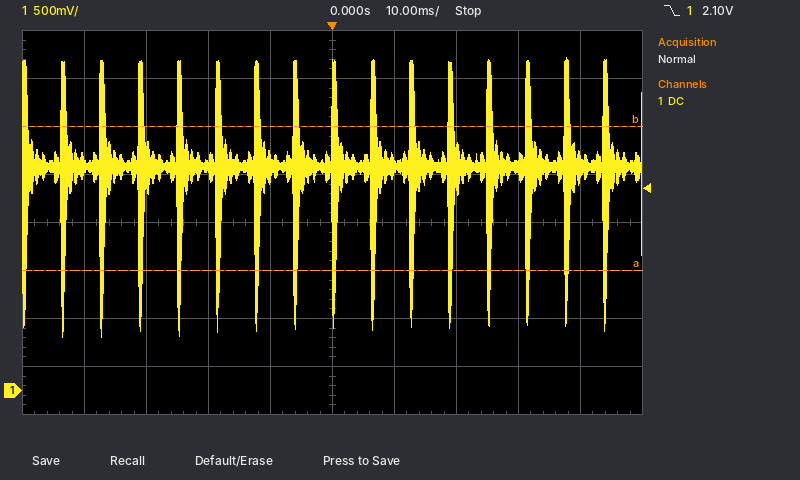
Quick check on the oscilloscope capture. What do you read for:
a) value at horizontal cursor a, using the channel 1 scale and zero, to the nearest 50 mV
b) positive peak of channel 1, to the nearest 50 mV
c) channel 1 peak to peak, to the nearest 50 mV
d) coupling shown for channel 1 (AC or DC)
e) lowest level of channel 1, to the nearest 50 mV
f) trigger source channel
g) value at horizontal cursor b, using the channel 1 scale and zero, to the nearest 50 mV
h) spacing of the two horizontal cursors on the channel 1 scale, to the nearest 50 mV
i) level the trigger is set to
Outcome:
1.25 V
3.45 V
2.90 V
DC
550 mV
channel 1
2.75 V
1.50 V
2.10 V
